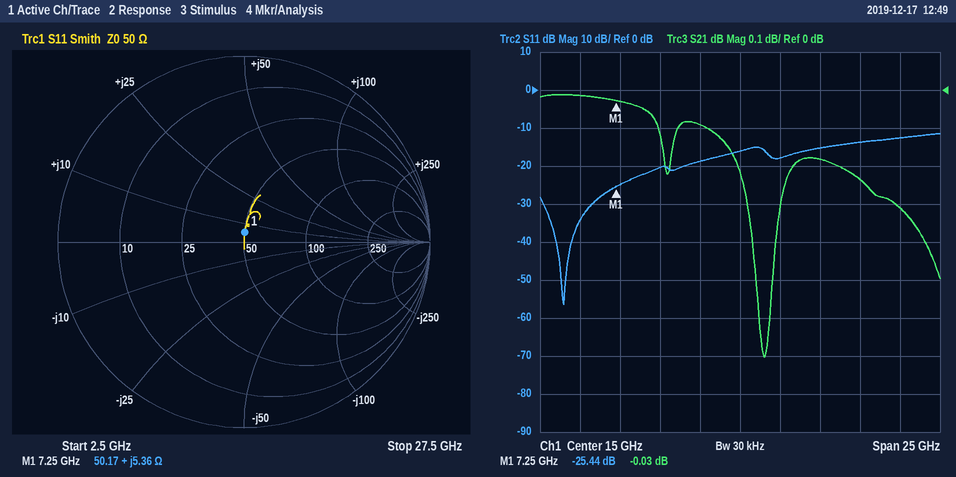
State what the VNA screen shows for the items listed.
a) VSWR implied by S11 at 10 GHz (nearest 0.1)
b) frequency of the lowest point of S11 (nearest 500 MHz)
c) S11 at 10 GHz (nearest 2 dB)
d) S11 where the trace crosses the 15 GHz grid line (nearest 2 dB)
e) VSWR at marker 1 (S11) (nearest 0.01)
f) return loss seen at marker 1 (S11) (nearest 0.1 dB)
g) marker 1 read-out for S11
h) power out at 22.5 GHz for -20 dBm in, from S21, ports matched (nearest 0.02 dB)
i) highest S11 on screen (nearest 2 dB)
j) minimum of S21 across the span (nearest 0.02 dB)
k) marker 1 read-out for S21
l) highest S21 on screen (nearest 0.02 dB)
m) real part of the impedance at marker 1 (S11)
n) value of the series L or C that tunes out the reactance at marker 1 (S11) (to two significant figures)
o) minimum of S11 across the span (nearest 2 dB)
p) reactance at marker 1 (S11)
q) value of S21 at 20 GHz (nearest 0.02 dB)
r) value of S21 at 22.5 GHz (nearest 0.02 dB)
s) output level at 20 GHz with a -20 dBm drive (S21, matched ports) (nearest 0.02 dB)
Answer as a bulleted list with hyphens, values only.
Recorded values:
- 1.2
- 4.0 GHz
- -20 dB
- -16 dB
- 1.11
- 25.4 dB
- -25.44 dB
- -20.24 dBm
- -12 dB
- -0.70 dB
- -0.03 dB
- -0.02 dB
- 50.17 Ω
- 4.1 pF
- -56 dB
- +5.36 Ω
- -0.18 dB
- -0.24 dB
- -20.18 dBm
